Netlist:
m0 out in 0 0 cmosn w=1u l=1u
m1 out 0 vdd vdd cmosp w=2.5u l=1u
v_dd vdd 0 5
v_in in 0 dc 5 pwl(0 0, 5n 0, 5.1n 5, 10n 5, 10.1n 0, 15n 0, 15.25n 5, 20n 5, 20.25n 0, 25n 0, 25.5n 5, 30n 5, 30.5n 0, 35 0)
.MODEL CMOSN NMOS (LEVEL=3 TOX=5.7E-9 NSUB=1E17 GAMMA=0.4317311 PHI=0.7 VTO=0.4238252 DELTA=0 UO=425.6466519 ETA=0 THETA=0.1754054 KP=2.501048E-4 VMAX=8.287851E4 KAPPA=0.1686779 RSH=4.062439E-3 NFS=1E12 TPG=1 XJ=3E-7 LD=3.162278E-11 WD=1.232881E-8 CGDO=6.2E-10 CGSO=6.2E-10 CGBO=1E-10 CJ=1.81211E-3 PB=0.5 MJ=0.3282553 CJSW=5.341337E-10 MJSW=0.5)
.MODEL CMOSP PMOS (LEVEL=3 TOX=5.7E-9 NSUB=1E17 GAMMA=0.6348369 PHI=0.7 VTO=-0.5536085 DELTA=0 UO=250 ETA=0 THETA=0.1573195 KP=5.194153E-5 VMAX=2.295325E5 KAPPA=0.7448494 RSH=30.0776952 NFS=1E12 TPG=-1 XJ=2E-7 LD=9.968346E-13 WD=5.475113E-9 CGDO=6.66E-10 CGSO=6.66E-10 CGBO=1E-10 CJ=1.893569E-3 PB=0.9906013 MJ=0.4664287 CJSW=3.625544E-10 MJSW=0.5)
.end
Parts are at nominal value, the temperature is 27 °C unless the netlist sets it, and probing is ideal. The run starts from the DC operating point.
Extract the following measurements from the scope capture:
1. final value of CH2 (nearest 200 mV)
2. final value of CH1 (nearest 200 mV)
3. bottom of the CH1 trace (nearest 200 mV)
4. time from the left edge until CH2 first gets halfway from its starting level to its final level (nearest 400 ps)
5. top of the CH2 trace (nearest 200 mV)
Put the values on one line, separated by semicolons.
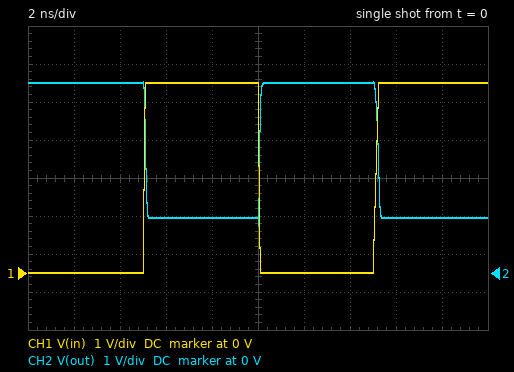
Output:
1.4 V; 5.0 V; 0 V; 5.2 ns; 5.0 V
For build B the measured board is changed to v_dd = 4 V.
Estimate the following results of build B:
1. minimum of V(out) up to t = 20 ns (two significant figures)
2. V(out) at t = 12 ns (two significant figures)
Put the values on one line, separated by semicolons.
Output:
490 mV; 4.0 V
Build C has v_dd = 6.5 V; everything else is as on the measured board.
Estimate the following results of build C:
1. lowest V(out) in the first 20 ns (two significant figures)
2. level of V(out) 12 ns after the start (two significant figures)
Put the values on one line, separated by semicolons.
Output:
4.0 V; 6.5 V
